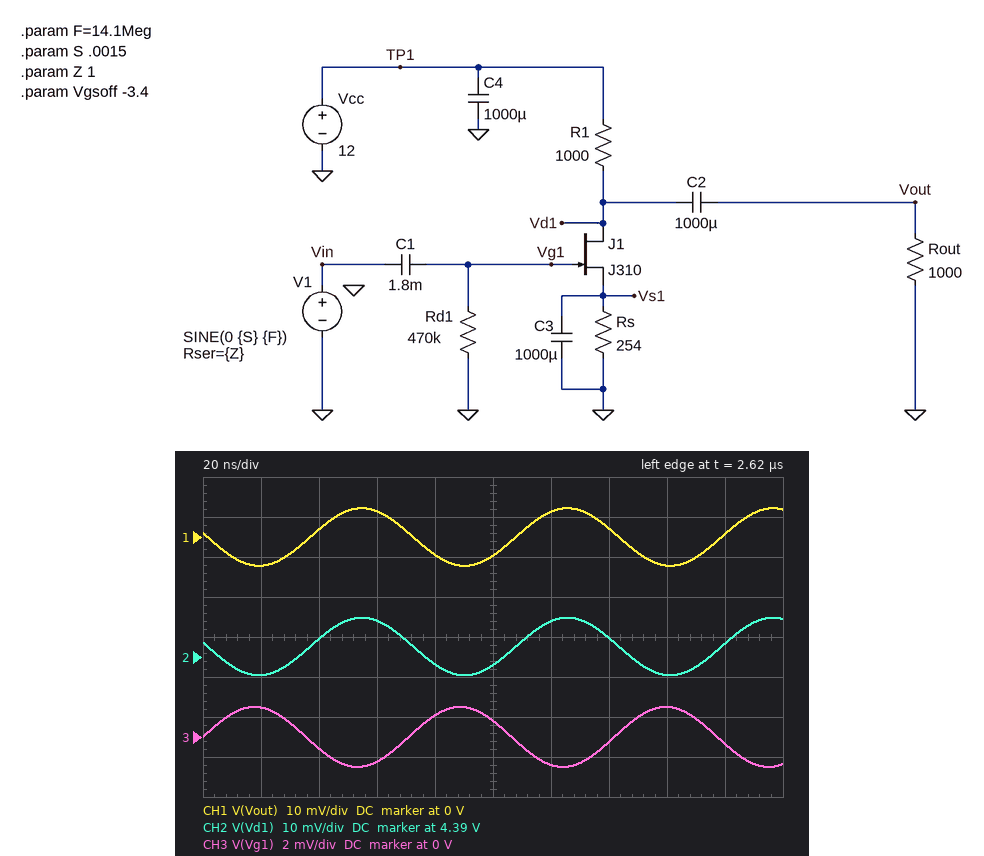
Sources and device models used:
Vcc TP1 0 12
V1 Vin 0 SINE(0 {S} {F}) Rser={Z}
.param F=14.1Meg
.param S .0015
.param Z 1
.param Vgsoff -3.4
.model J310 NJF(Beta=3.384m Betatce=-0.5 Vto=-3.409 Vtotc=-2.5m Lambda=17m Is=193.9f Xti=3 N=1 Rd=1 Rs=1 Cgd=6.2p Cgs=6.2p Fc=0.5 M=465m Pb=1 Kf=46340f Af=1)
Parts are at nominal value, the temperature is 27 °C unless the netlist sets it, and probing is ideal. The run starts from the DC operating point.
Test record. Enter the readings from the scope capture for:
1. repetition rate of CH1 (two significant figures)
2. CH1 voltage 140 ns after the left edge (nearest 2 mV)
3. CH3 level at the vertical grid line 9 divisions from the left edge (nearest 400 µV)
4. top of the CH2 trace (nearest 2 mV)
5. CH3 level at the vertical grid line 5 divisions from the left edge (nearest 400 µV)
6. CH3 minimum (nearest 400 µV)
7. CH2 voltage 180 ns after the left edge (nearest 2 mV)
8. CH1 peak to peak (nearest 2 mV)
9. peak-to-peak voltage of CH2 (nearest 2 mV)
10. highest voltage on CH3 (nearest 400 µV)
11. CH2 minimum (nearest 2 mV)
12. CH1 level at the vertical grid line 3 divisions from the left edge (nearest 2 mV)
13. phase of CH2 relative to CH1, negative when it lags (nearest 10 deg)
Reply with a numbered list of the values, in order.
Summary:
1. 14 MHz
2. 2 mV
3. -400 µV
4. 4.400 V
5. 800 µV
6. -1.6 mV
7. 4.394 V
8. 14 mV
9. 14 mV
10. 1.6 mV
11. 4.386 V
12. 6 mV
13. 0 deg
